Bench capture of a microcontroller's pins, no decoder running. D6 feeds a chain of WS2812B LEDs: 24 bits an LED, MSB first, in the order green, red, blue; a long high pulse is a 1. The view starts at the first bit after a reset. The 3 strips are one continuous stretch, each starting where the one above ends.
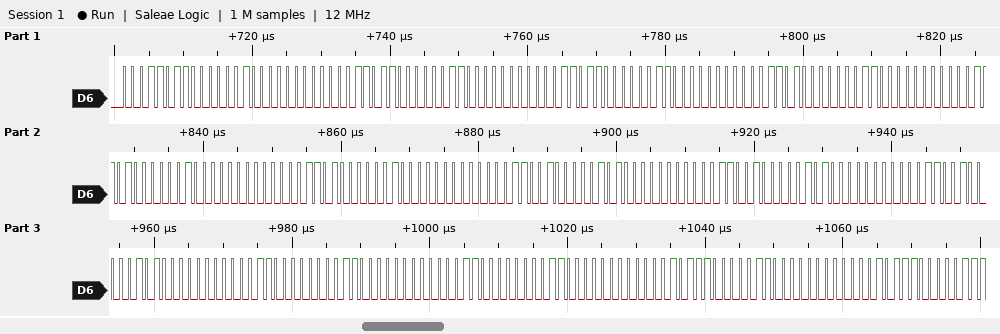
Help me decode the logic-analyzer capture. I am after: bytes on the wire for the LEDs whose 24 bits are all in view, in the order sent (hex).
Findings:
1B 02 00 1B 03 00 1B 03 00 1A 03 00 1A 04 00 1A 04 00 19 05 00 19 05 00 19 05 00 18 06 00 18 06 00 17 06 00
